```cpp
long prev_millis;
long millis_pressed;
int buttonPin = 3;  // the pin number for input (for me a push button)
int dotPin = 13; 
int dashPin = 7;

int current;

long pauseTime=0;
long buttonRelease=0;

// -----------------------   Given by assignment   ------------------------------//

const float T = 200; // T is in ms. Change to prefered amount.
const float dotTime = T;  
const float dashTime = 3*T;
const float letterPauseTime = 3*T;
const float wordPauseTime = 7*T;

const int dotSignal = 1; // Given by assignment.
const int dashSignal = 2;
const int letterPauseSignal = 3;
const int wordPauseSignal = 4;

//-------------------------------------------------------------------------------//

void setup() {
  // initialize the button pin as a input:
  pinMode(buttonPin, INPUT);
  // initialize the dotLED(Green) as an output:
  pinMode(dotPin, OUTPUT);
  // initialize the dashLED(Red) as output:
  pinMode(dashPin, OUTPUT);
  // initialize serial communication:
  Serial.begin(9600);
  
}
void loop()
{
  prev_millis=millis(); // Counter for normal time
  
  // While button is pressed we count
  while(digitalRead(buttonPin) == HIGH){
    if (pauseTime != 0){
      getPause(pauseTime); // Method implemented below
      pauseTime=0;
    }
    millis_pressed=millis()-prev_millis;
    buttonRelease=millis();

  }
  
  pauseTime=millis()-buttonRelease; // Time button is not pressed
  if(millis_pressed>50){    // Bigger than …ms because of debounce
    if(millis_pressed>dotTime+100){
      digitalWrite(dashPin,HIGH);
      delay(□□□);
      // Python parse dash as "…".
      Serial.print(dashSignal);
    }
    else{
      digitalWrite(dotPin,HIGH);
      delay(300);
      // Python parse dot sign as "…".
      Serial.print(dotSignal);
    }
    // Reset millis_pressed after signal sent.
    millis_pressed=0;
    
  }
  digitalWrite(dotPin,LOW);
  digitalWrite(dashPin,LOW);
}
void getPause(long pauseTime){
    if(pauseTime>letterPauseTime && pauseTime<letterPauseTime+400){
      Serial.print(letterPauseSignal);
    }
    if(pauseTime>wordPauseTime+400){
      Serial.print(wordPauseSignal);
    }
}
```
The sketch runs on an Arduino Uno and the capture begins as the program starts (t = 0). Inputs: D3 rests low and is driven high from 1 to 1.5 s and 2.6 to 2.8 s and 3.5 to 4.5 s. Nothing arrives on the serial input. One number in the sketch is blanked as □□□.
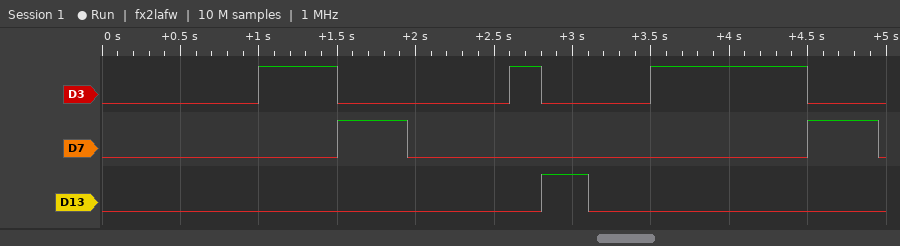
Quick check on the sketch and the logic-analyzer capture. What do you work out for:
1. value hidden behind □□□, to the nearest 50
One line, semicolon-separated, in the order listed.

450
